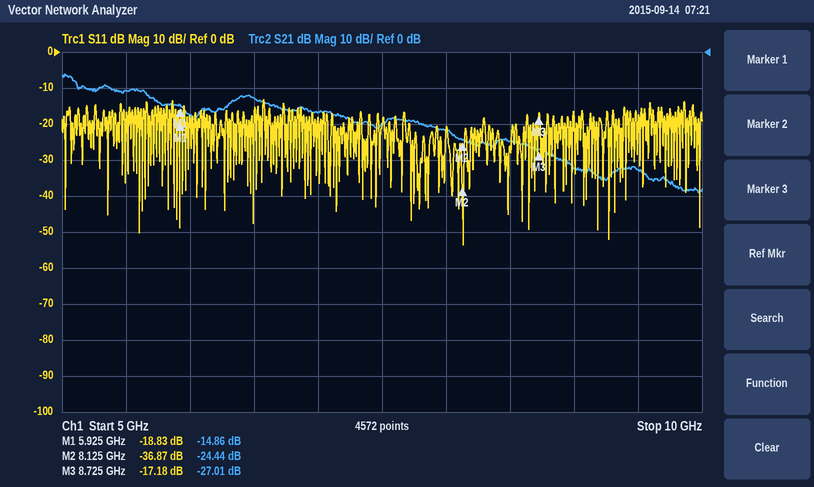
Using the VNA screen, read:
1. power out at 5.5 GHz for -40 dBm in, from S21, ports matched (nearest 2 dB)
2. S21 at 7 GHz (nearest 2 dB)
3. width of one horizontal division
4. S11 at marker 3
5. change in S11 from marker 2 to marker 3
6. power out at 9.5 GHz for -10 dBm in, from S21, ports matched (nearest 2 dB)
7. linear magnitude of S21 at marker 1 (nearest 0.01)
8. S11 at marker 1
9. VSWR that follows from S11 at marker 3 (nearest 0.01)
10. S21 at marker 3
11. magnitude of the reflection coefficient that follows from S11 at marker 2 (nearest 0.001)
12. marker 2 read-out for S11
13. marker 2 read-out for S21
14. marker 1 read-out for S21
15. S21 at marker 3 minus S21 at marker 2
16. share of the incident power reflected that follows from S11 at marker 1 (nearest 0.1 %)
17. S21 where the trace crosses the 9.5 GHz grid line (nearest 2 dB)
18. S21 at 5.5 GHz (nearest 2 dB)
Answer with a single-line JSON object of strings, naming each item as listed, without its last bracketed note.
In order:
{"power out at 5.5 GHz for -40 dBm in, from S21, ports matched": "-50 dBm", "S21 at 7 GHz": "-16 dB", "width of one horizontal division": "500 MHz", "S11 at marker 3": "-17.18 dB", "change in S11 from marker 2 to marker 3": "19.69 dB", "power out at 9.5 GHz for -10 dBm in, from S21, ports matched": "-42 dBm", "linear magnitude of S21 at marker 1": "0.18", "S11 at marker 1": "-18.83 dB", "VSWR that follows from S11 at marker 3": "1.32", "S21 at marker 3": "-27.01 dB", "magnitude of the reflection coefficient that follows from S11 at marker 2": "0.014", "marker 2 read-out for S11": "-36.87 dB", "marker 2 read-out for S21": "-24.44 dB", "marker 1 read-out for S21": "-14.86 dB", "S21 at marker 3 minus S21 at marker 2": "-2.57 dB", "share of the incident power reflected that follows from S11 at marker 1": "1.3 %", "S21 where the trace crosses the 9.5 GHz grid line": "-32 dB", "S21 at 5.5 GHz": "-10 dB"}
